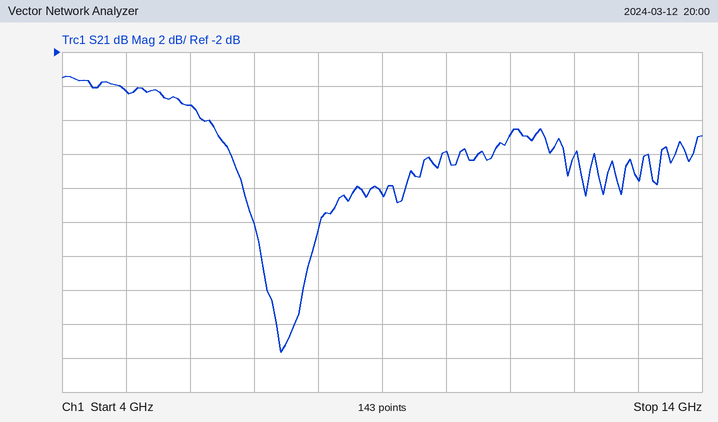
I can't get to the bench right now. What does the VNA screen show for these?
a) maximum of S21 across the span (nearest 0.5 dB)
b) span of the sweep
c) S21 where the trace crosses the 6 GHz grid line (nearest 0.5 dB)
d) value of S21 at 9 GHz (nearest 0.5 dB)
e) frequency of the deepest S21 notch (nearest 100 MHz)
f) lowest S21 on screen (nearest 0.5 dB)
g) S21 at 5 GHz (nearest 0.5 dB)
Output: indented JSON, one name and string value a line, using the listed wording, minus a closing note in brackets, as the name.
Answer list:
{
  "maximum of S21 across the span": "-3.5 dB",
  "span of the sweep": "10 GHz",
  "S21 where the trace crosses the 6 GHz grid line": "-5.0 dB",
  "value of S21 at 9 GHz": "-10.5 dB",
  "frequency of the deepest S21 notch": "7.4 GHz",
  "lowest S21 on screen": "-19.5 dB",
  "S21 at 5 GHz": "-4.5 dB"
}
